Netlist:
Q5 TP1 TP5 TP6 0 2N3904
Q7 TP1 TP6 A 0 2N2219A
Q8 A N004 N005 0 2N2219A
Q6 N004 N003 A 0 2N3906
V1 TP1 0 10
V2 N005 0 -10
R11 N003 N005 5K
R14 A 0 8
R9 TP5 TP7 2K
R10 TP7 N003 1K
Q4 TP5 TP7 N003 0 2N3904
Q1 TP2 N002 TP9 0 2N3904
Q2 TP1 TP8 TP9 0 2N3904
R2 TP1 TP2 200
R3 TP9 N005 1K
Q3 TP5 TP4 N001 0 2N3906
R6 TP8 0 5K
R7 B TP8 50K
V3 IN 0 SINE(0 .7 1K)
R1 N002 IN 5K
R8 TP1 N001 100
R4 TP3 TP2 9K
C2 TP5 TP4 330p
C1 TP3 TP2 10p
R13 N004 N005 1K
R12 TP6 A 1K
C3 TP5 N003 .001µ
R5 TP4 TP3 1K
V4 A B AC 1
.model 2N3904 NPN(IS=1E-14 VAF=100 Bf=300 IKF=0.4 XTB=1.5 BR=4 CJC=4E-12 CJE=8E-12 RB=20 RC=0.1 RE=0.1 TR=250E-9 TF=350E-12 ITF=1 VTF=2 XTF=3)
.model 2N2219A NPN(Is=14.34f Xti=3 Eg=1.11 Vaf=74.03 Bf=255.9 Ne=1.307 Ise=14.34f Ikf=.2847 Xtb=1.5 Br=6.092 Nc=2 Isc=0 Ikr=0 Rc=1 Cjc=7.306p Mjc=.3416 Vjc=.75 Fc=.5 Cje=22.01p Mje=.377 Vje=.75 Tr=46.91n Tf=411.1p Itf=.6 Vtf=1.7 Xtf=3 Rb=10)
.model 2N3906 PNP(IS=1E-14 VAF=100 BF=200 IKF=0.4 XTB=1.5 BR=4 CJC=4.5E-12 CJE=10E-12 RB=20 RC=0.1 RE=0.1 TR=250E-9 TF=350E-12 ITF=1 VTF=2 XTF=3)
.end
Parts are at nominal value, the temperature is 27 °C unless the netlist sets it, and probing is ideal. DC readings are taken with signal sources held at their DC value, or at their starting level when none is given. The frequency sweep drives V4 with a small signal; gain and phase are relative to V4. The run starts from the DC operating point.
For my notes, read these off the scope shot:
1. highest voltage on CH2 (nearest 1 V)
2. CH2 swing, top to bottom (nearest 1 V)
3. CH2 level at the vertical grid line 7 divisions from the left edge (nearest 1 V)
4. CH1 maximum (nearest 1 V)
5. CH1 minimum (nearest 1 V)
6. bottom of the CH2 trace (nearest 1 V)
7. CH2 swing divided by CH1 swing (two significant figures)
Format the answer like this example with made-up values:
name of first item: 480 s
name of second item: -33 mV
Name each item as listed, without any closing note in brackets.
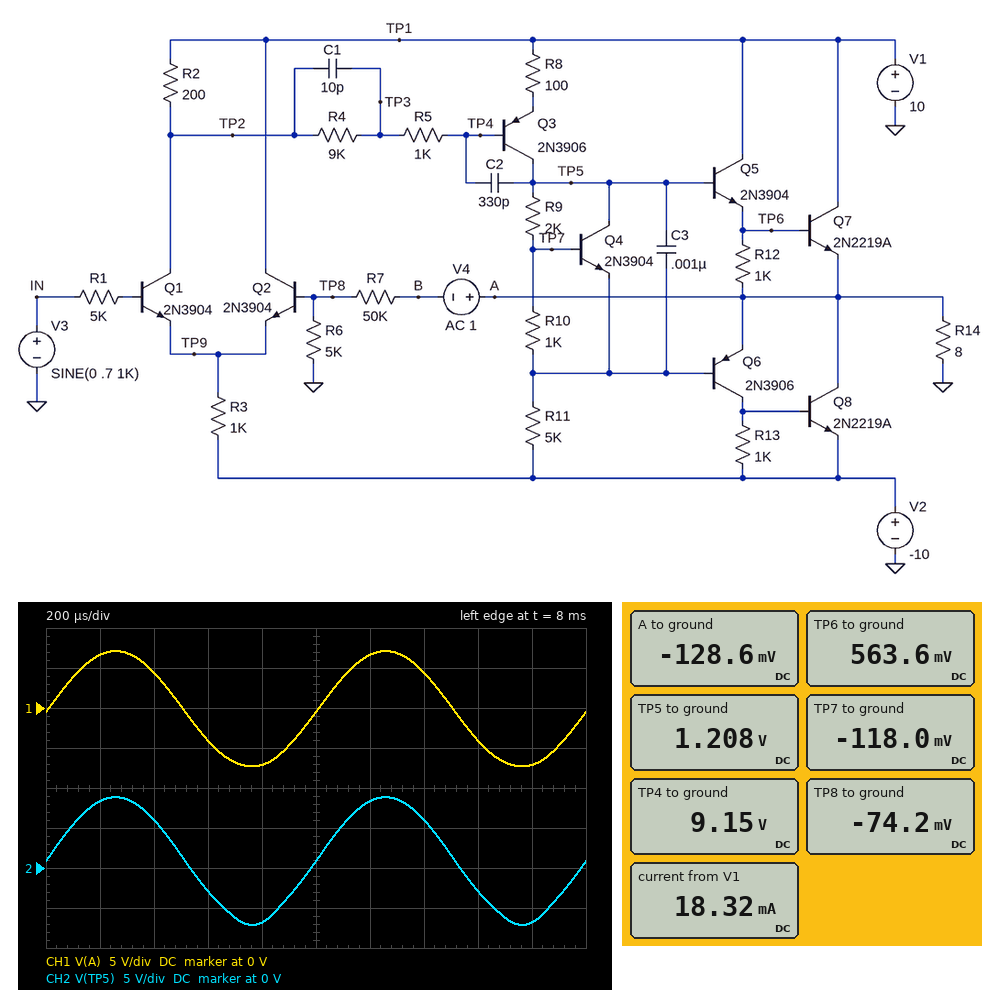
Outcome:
highest voltage on CH2: 9 V
CH2 swing, top to bottom: 16 V
CH2 level at the vertical grid line 7 divisions from the left edge: 6 V
CH1 maximum: 7 V
CH1 minimum: -7 V
bottom of the CH2 trace: -7 V
CH2 swing divided by CH1 swing: 1.1
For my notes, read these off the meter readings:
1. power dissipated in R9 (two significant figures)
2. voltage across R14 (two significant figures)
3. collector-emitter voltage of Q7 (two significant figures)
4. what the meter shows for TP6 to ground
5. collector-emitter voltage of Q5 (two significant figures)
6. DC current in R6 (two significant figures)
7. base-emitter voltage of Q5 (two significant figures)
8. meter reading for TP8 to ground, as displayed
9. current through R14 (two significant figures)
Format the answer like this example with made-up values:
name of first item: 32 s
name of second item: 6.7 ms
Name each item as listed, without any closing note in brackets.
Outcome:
power dissipated in R9: 880 µW
voltage across R14: 130 mV
collector-emitter voltage of Q7: 10 V
what the meter shows for TP6 to ground: 563.6 mV
collector-emitter voltage of Q5: 9.4 V
DC current in R6: 15 µA
base-emitter voltage of Q5: 640 mV
meter reading for TP8 to ground, as displayed: -74.2 mV
current through R14: 16 mA
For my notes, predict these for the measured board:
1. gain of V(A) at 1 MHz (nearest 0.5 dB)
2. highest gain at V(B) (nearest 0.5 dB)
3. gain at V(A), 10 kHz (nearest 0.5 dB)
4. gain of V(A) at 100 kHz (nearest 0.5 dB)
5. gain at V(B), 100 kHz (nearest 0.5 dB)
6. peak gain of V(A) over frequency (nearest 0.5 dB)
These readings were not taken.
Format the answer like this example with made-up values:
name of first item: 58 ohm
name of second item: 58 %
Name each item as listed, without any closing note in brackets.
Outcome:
gain of V(A) at 1 MHz: -35.5 dB
highest gain at V(B): 0 dB
gain at V(A), 10 kHz: -1.5 dB
gain of V(A) at 100 kHz: -14.5 dB
gain at V(B), 100 kHz: 0 dB
peak gain of V(A) over frequency: -0.5 dB
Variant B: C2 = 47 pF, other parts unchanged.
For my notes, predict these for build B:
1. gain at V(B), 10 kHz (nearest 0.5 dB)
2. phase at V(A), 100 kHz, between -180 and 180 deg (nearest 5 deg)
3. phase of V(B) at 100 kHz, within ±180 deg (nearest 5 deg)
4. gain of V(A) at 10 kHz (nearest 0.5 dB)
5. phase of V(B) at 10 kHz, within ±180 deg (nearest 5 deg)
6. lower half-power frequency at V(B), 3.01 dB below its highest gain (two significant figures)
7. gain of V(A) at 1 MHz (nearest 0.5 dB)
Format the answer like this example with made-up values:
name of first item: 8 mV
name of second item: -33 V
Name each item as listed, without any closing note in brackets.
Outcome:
gain at V(B), 10 kHz: -19.5 dB
phase at V(A), 100 kHz, between -180 and 180 deg: -35 deg
phase of V(B) at 100 kHz, within ±180 deg: -130 deg
gain of V(A) at 10 kHz: -0.5 dB
phase of V(B) at 10 kHz, within ±180 deg: -140 deg
lower half-power frequency at V(B), 3.01 dB below its highest gain: 140 kHz
gain of V(A) at 1 MHz: -19.0 dB
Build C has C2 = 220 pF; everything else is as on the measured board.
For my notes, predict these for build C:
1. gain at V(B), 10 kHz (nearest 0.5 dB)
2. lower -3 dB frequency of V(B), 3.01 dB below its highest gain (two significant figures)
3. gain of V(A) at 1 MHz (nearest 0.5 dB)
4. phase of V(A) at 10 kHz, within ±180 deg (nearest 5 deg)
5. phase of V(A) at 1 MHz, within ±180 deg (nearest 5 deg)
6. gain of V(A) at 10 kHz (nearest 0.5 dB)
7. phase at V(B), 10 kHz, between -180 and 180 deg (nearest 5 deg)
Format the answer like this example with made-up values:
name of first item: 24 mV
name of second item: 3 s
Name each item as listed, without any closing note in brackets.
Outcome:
gain at V(B), 10 kHz: -10.0 dB
lower -3 dB frequency of V(B), 3.01 dB below its highest gain: 31 kHz
gain of V(A) at 1 MHz: -32.0 dB
phase of V(A) at 10 kHz, within ±180 deg: -20 deg
phase of V(A) at 1 MHz, within ±180 deg: -115 deg
gain of V(A) at 10 kHz: -1.0 dB
phase at V(B), 10 kHz, between -180 and 180 deg: -120 deg
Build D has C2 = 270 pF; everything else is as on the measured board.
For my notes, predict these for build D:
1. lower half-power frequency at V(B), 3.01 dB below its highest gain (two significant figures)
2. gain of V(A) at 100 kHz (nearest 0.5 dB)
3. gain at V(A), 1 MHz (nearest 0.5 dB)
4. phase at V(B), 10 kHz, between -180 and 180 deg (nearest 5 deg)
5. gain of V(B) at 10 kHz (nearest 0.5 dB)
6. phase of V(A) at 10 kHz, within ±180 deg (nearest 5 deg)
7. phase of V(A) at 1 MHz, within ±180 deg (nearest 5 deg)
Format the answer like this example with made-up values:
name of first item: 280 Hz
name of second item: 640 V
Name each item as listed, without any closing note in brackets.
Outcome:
lower half-power frequency at V(B), 3.01 dB below its highest gain: 25 kHz
gain of V(A) at 100 kHz: -13.0 dB
gain at V(A), 1 MHz: -34.0 dB
phase at V(B), 10 kHz, between -180 and 180 deg: -120 deg
gain of V(B) at 10 kHz: -8.5 dB
phase of V(A) at 10 kHz, within ±180 deg: -20 deg
phase of V(A) at 1 MHz, within ±180 deg: -115 deg
